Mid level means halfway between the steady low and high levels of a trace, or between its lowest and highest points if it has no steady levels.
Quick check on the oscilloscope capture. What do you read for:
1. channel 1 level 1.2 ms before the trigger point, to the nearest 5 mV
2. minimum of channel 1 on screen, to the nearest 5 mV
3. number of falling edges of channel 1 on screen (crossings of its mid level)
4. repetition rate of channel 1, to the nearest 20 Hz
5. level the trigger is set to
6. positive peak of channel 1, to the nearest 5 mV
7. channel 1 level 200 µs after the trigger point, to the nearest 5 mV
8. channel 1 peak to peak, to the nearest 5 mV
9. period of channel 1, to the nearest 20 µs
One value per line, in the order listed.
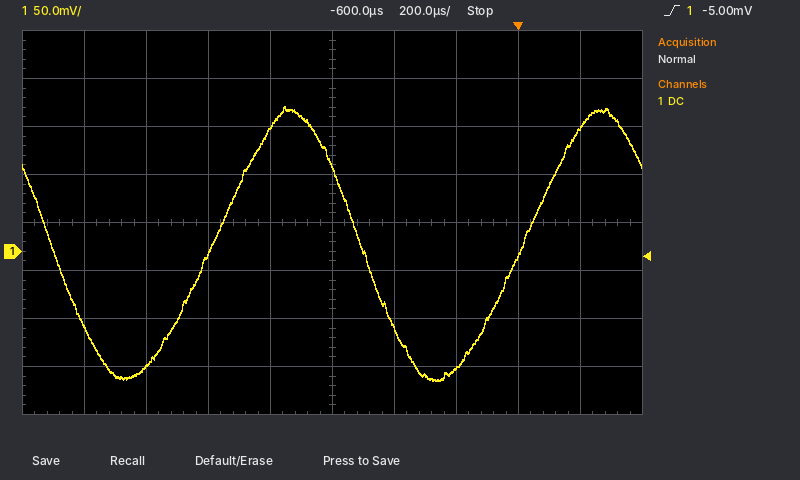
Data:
-120 mV
-135 mV
2
1.00 kHz
-5.00 mV
150 mV
130 mV
285 mV
1.00 ms
